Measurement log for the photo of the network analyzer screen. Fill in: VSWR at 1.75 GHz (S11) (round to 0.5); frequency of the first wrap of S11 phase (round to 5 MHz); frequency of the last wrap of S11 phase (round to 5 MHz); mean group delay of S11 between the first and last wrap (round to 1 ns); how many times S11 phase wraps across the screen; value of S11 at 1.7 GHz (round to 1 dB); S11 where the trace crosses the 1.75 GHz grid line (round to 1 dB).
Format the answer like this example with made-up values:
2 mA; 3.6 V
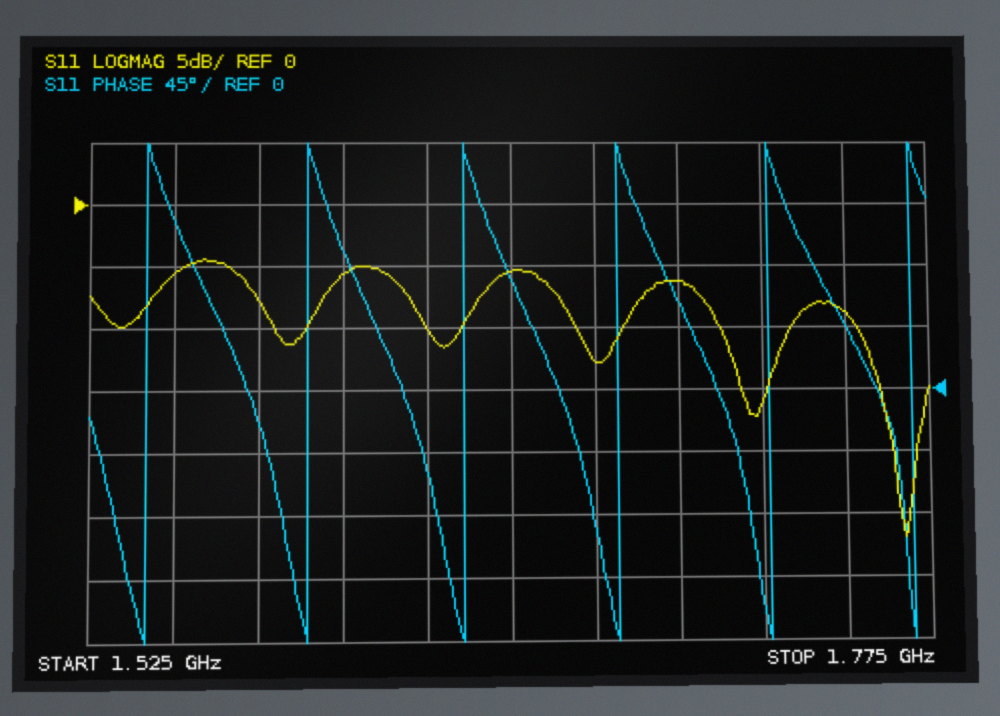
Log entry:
2.0; 1.540 GHz; 1.770 GHz; 22 ns; 6; -6 dB; -9 dB
